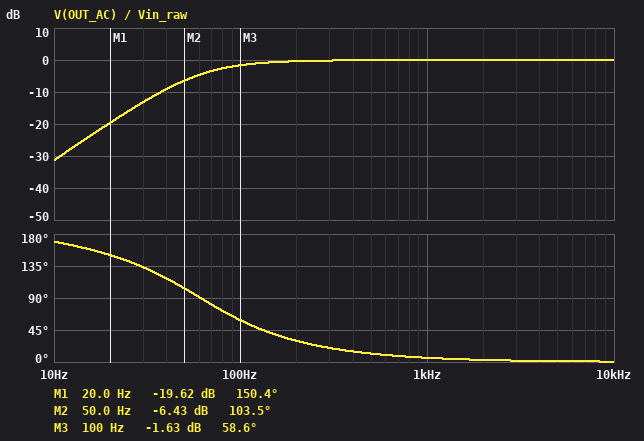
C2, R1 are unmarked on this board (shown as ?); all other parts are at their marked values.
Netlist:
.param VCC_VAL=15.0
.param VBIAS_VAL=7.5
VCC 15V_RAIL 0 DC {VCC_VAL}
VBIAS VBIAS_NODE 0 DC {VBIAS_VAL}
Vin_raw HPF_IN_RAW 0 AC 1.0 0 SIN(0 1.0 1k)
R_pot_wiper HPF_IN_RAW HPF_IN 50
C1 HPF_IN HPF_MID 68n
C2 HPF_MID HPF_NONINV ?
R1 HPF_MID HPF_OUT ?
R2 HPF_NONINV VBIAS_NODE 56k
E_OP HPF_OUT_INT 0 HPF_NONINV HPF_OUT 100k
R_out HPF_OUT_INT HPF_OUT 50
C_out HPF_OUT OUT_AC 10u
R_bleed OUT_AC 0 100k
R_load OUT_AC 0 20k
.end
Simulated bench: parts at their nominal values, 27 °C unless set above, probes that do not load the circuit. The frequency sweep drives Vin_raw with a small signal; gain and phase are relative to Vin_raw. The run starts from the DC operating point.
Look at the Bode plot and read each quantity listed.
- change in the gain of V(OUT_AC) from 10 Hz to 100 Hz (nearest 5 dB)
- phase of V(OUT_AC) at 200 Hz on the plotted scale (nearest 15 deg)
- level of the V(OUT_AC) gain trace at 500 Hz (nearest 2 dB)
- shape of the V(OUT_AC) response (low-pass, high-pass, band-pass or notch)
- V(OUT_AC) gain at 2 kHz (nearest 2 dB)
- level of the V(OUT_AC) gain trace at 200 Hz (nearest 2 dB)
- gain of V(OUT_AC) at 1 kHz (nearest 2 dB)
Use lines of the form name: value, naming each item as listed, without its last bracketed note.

change in the gain of V(OUT_AC) from 10 Hz to 100 Hz: 30 dB
phase of V(OUT_AC) at 200 Hz on the plotted scale: 30 deg
level of the V(OUT_AC) gain trace at 500 Hz: 0 dB
shape of the V(OUT_AC) response: high-pass
V(OUT_AC) gain at 2 kHz: 0 dB
level of the V(OUT_AC) gain trace at 200 Hz: 0 dB
gain of V(OUT_AC) at 1 kHz: 0 dB
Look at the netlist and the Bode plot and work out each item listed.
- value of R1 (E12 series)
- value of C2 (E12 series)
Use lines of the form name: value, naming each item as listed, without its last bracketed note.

value of R1: 39 kΩ
value of C2: 47 nF
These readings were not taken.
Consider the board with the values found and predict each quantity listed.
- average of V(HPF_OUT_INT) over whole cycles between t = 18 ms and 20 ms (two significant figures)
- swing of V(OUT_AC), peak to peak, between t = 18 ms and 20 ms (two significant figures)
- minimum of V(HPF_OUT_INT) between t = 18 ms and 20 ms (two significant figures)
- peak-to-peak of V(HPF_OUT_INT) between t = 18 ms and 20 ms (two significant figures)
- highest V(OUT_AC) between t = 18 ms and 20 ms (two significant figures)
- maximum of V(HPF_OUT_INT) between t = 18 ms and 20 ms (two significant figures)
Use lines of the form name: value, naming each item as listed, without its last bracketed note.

average of V(HPF_OUT_INT) over whole cycles between t = 18 ms and 20 ms: 7.5 V
swing of V(OUT_AC), peak to peak, between t = 18 ms and 20 ms: 2.0 V
minimum of V(HPF_OUT_INT) between t = 18 ms and 20 ms: 6.5 V
peak-to-peak of V(HPF_OUT_INT) between t = 18 ms and 20 ms: 2.0 V
highest V(OUT_AC) between t = 18 ms and 20 ms: 1.0 V
maximum of V(HPF_OUT_INT) between t = 18 ms and 20 ms: 8.5 V
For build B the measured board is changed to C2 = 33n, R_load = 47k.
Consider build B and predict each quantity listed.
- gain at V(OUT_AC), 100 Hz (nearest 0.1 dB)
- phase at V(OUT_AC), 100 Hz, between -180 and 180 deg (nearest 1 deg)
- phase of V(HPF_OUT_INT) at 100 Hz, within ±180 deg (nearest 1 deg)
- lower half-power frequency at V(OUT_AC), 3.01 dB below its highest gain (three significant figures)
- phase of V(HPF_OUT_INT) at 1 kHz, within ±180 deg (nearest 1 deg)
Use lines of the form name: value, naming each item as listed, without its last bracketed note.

gain at V(OUT_AC), 100 Hz: -2.7 dB
phase at V(OUT_AC), 100 Hz, between -180 and 180 deg: 70 deg
phase of V(HPF_OUT_INT) at 100 Hz, within ±180 deg: 69 deg
lower half-power frequency at V(OUT_AC), 3.01 dB below its highest gain: 94.9 Hz
phase of V(HPF_OUT_INT) at 1 kHz, within ±180 deg: 7 deg
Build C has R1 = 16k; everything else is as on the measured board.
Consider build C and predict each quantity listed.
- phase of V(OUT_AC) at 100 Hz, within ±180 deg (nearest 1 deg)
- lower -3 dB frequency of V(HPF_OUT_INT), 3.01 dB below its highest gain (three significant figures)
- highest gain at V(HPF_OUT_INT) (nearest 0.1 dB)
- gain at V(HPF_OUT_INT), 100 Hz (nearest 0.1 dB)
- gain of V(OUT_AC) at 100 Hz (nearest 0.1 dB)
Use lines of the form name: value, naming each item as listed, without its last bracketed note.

phase of V(OUT_AC) at 100 Hz, within ±180 deg: 84 deg
lower -3 dB frequency of V(HPF_OUT_INT), 3.01 dB below its highest gain: 81.8 Hz
highest gain at V(HPF_OUT_INT): 0.8 dB
gain at V(HPF_OUT_INT), 100 Hz: -0.2 dB
gain of V(OUT_AC) at 100 Hz: -0.3 dB
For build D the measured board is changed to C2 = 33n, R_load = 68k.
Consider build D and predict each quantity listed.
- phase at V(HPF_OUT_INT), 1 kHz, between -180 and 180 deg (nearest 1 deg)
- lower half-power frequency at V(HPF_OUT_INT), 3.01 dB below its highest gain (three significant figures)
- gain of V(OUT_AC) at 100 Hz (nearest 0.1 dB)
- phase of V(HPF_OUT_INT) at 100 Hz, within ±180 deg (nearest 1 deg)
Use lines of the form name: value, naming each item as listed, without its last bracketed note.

phase at V(HPF_OUT_INT), 1 kHz, between -180 and 180 deg: 7 deg
lower half-power frequency at V(HPF_OUT_INT), 3.01 dB below its highest gain: 94.9 Hz
gain of V(OUT_AC) at 100 Hz: -2.7 dB
phase of V(HPF_OUT_INT) at 100 Hz, within ±180 deg: 69 deg
